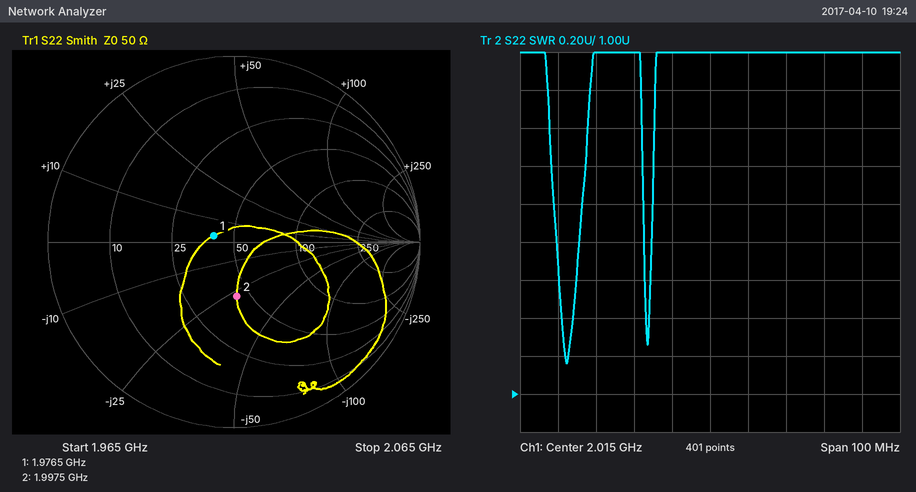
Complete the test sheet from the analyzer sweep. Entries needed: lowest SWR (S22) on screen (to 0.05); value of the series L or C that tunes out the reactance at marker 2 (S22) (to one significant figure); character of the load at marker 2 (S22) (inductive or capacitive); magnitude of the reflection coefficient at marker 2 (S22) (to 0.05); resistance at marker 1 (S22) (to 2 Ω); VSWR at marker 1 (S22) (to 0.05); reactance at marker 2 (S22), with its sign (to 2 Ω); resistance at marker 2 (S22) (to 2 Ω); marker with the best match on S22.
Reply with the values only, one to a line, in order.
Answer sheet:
1.15
2 nH
capacitive
0.30
40 Ω
1.25
-28 Ω
44 Ω
marker 1
